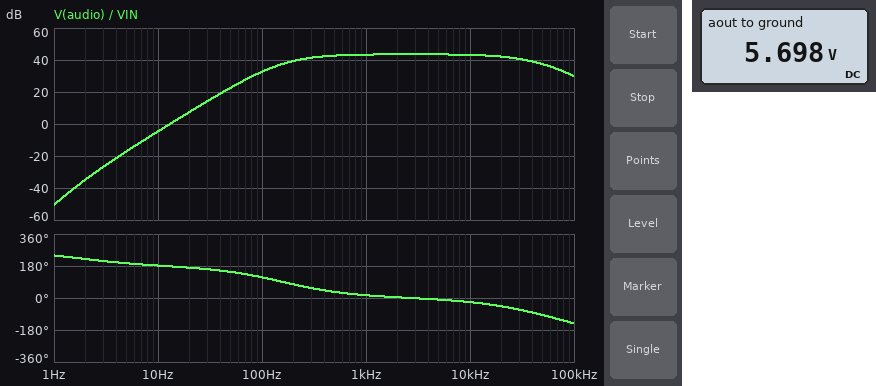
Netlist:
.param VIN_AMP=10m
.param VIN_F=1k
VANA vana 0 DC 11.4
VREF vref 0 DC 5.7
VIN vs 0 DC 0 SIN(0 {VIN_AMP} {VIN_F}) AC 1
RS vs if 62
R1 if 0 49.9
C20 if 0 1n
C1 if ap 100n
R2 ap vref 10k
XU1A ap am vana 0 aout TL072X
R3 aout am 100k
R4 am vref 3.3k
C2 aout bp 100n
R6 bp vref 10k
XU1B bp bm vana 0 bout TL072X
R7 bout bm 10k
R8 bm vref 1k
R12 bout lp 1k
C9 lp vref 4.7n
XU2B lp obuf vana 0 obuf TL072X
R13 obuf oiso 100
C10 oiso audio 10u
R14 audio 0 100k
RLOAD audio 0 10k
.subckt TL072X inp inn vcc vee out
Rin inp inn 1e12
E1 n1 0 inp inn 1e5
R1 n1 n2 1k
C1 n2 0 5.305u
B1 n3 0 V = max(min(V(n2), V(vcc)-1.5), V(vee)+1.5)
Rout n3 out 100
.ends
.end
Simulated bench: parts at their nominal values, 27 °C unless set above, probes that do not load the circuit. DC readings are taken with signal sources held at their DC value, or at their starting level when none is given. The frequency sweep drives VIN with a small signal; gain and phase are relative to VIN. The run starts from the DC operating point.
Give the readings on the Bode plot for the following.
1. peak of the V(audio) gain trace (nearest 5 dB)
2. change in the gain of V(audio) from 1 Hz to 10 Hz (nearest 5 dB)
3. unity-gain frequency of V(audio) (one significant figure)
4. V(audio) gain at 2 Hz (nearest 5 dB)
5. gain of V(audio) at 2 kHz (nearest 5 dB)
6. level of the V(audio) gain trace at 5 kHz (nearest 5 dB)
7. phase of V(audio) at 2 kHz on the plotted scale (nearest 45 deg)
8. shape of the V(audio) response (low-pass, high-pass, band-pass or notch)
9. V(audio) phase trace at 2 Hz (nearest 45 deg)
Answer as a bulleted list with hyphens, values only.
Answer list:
- 45 dB
- 45 dB
- 10 Hz
- -35 dB
- 45 dB
- 45 dB
- 0 deg
- band-pass
- 225 deg
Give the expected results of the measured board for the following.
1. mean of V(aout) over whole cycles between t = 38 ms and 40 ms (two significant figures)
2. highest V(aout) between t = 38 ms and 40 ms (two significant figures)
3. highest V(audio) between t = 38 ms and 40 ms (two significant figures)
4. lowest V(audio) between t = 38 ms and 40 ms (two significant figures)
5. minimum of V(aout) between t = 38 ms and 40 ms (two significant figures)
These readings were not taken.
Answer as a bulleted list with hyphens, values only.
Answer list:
- 5.7 V
- 5.8 V
- 1.5 V
- -1.5 V
- 5.6 V
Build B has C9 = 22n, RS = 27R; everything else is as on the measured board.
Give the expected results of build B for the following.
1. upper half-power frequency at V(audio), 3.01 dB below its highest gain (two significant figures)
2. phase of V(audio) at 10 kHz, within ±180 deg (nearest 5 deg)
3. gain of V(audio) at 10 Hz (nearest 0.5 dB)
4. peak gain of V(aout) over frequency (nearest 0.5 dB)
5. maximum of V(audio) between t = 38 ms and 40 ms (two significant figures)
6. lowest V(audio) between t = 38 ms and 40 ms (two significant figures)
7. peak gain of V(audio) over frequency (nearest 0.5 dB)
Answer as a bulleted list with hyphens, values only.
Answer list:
- 7.6 kHz
- -60 deg
- -1.5 dB
- 26.0 dB
- 2.1 V
- -2.1 V
- 46.5 dB
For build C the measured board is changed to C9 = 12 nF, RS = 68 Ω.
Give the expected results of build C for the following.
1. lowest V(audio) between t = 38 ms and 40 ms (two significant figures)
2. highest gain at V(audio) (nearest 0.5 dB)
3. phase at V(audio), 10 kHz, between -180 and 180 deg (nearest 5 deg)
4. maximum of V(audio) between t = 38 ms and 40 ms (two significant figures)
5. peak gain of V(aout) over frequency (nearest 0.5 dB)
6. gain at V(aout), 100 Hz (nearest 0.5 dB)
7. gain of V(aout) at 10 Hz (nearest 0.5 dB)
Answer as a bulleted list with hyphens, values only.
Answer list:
- -1.4 V
- 43.0 dB
- -45 deg
- 1.4 V
- 22.5 dB
- 17.0 dB
- -1.5 dB
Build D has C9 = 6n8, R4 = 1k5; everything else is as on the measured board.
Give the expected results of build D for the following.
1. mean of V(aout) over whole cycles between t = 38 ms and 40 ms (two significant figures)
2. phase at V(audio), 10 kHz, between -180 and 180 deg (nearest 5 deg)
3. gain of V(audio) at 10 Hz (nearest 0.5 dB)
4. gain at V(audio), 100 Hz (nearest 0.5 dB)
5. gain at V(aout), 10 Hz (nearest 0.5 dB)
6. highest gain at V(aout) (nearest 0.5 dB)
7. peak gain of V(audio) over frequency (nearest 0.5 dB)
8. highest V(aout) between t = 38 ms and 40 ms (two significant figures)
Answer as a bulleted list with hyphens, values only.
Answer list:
- 5.7 V
- -35 deg
- 2.0 dB
- 39.5 dB
- 5.5 dB
- 29.5 dB
- 50.0 dB
- 6.0 V
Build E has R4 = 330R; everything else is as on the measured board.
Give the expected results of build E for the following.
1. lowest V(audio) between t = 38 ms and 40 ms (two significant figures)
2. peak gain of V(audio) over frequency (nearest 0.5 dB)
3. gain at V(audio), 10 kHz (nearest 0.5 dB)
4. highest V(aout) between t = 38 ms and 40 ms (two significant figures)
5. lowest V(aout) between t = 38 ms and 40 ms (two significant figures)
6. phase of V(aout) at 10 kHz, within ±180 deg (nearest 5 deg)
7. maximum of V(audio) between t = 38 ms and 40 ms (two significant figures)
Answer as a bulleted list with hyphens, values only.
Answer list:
- -4.1 V
- 63.0 dB
- 60.0 dB
- 7.0 V
- 4.4 V
- -45 deg
- 4.1 V
